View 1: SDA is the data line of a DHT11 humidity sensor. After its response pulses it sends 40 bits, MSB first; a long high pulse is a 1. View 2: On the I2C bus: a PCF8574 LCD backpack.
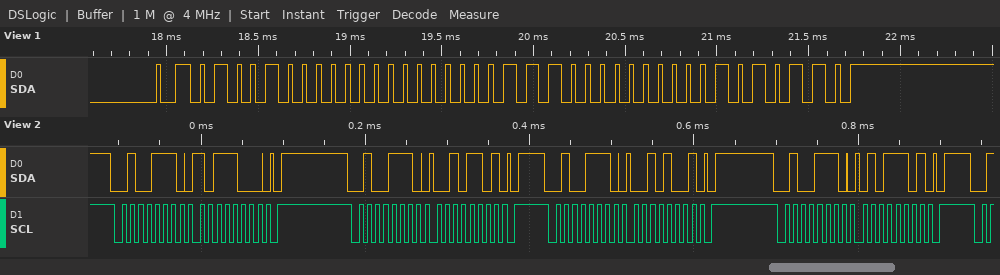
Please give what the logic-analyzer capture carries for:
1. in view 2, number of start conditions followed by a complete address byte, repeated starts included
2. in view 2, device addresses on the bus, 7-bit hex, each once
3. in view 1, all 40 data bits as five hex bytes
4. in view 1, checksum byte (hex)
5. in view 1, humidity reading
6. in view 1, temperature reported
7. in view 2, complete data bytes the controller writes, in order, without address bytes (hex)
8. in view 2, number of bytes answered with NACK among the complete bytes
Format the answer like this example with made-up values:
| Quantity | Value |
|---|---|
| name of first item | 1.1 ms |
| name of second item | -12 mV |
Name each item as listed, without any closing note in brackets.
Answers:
| Quantity | Value |
|---|---|
| in view 2, number of start conditions followed by a complete address byte, repeated starts included | 4 |
| in view 2, device addresses on the bus, 7-bit hex, each once | 0x27 |
| in view 1, all 40 data bits as five hex bytes | 48 00 0E 00 56 |
| in view 1, checksum byte | 0x56 |
| in view 1, humidity reading | 72 % |
| in view 1, temperature reported | 14.0 °C |
| in view 2, complete data bytes the controller writes, in order, without address bytes | B8 2D 29 5D |
| in view 2, number of bytes answered with NACK among the complete bytes | 0 |
